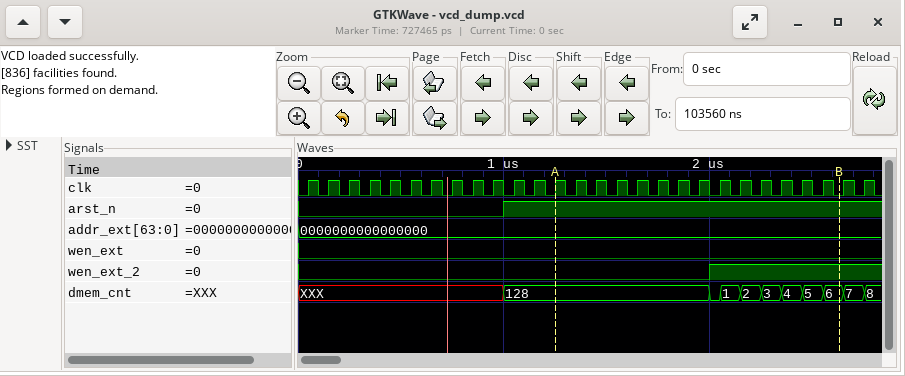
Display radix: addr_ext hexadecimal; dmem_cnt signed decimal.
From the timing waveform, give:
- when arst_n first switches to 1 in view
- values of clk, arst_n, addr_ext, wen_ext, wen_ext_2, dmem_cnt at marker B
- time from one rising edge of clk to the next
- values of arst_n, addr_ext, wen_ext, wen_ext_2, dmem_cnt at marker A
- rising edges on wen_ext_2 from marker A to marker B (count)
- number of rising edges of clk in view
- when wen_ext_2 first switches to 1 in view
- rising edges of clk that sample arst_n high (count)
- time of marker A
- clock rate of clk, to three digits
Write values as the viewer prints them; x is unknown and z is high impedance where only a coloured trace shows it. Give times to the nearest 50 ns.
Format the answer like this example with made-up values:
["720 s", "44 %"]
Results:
["1000 ns", "clk=0, arst_n=1, addr_ext=0000000000000000, wen_ext=0, wen_ext_2=1, dmem_cnt=6", "100 ns", "arst_n=1, addr_ext=0000000000000000, wen_ext=0, wen_ext_2=0, dmem_cnt=128", "1", "28", "2000 ns", "18", "1250 ns", "10.0 MHz"]
